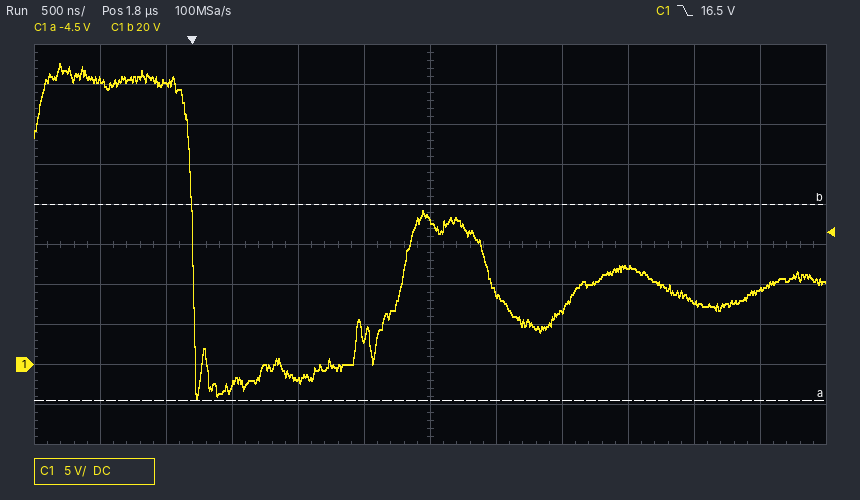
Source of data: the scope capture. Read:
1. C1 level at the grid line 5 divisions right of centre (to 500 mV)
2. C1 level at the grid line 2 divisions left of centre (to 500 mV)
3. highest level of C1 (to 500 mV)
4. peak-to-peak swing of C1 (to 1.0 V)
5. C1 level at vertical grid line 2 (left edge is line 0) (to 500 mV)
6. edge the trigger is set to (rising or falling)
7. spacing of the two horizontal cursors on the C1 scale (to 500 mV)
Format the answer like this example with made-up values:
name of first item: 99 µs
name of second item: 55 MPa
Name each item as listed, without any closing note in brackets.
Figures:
C1 level at the grid line 5 divisions right of centre: 9.5 V
C1 level at the grid line 2 divisions left of centre: -2.0 V
highest level of C1: 37.5 V
peak-to-peak swing of C1: 42.0 V
C1 level at vertical grid line 2 (left edge is line 0): 35.0 V
edge the trigger is set to: falling
spacing of the two horizontal cursors on the C1 scale: 24.5 V
